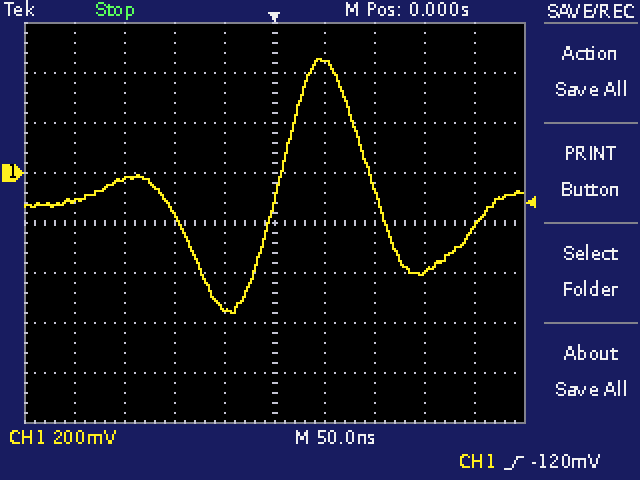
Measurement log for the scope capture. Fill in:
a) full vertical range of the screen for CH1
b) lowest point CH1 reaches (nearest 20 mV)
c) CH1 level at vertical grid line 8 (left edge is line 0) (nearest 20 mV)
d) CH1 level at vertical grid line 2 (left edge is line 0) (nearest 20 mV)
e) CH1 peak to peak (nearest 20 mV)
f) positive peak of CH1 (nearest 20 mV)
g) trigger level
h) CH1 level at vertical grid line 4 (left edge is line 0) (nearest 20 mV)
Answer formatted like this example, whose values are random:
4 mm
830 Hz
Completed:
1.6 V
-560 mV
-400 mV
-20 mV
1.02 V
460 mV
-120 mV
-540 mV
